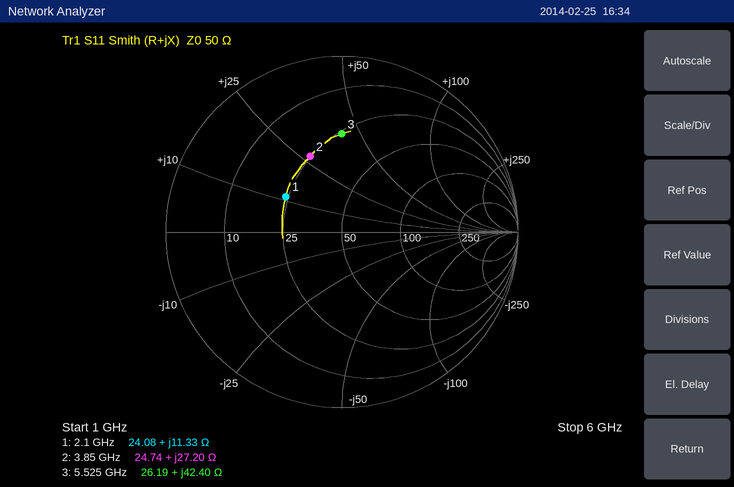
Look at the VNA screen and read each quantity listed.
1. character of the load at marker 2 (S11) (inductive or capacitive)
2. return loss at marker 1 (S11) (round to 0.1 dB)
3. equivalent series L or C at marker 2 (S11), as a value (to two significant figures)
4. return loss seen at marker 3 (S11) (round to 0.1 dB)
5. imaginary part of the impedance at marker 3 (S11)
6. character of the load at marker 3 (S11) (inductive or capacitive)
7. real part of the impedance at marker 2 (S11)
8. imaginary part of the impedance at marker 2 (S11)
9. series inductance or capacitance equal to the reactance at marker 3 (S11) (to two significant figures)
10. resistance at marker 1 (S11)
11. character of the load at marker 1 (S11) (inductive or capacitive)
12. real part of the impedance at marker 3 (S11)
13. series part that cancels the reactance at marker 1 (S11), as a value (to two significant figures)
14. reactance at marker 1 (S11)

inductive
8.5 dB
1.1 nH
5.1 dB
+42.40 Ω
inductive
24.74 Ω
+27.20 Ω
1.2 nH
24.08 Ω
inductive
26.19 Ω
6.7 pF
+11.33 Ω
